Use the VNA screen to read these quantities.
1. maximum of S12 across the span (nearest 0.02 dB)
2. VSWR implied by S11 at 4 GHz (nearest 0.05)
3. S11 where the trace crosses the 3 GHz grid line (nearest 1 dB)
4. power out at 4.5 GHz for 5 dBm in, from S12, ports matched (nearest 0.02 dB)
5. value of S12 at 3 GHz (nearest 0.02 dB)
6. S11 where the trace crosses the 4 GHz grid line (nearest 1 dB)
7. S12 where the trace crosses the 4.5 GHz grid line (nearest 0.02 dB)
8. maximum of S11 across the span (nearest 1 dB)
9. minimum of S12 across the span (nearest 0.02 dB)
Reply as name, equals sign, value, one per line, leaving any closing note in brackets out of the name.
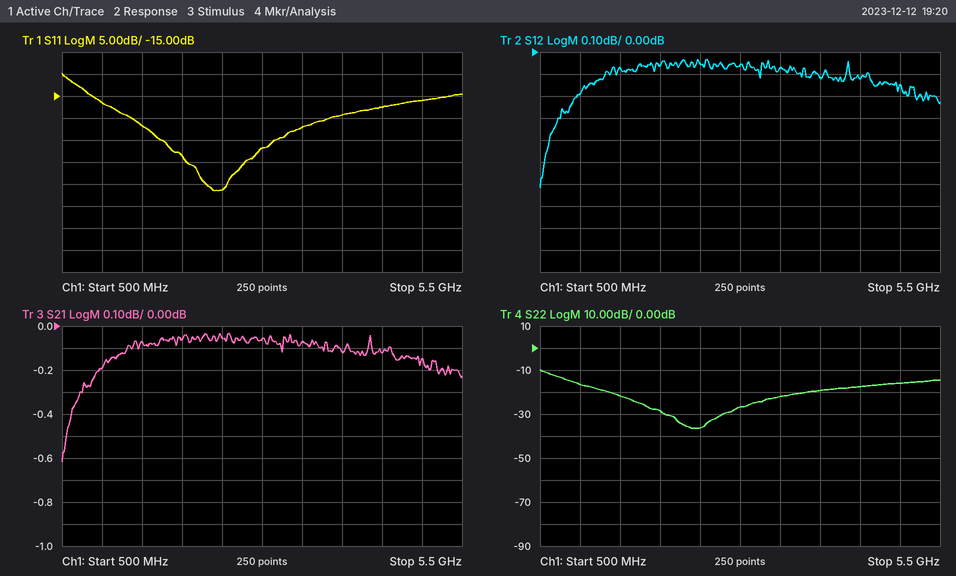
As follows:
maximum of S12 across the span = -0.04 dB
VSWR implied by S11 at 4 GHz = 1.25
S11 where the trace crosses the 3 GHz grid line = -27 dB
power out at 4.5 GHz for 5 dBm in, from S12, ports matched = 4.88 dBm
value of S12 at 3 GHz = -0.06 dB
S11 where the trace crosses the 4 GHz grid line = -19 dB
S12 where the trace crosses the 4.5 GHz grid line = -0.12 dB
maximum of S11 across the span = -10 dB
minimum of S12 across the span = -0.62 dB
